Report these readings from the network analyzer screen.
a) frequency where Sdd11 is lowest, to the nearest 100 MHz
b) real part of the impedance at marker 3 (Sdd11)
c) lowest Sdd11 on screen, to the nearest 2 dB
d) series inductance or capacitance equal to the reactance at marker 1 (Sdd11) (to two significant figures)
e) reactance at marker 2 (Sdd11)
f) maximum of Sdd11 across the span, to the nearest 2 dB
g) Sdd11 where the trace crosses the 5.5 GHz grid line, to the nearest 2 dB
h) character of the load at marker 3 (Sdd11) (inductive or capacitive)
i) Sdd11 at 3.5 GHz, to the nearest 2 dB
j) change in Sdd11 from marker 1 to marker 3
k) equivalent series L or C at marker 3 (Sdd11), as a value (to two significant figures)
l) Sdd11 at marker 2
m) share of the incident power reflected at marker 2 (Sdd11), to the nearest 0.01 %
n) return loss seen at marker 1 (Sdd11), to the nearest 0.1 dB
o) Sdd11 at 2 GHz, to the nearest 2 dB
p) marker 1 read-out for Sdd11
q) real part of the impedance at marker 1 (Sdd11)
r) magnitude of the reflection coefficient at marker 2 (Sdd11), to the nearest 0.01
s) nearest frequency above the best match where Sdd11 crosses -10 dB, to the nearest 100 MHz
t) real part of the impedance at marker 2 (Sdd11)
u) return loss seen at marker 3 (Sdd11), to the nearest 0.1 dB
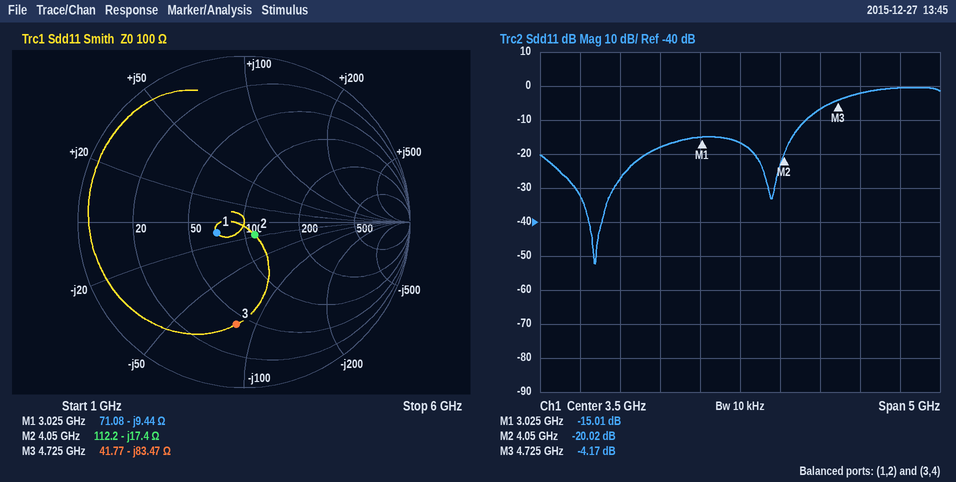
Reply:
1.7 GHz
41.77 Ω
-52 dB
5.6 pF
-17.4 Ω
0 dB
0 dB
capacitive
-16 dB
10.84 dB
400 fF
-20.02 dB
1.00 %
15.0 dB
-28 dB
-15.01 dB
71.08 Ω
0.10
4.3 GHz
112.2 Ω
4.2 dB
